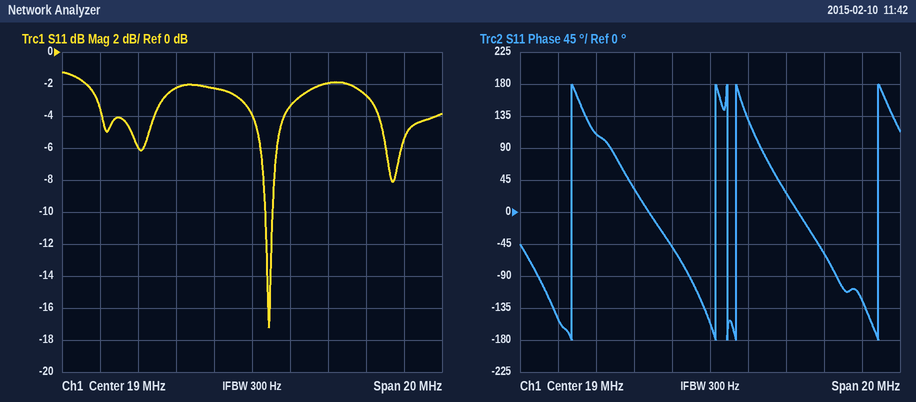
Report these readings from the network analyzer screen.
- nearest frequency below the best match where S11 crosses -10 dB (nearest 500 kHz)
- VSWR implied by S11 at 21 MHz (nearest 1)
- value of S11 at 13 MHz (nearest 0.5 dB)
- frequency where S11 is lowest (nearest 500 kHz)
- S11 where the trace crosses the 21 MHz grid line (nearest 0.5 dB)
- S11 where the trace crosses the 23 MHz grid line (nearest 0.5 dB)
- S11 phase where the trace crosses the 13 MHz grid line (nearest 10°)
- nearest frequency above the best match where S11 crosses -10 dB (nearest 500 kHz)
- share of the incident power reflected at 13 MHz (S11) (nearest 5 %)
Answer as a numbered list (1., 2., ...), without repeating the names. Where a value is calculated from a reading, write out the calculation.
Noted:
1. 19.5 MHz
2. |Γ| = 10^(-3.5/20) = 0.6683; VSWR = (1 + 0.6683)/(1 − 0.6683) ≈ 5
3. -6.0 dB
4. 20.0 MHz
5. -3.5 dB
6. -2.0 dB
7. 110°
8. 20.0 MHz
9. 10^(-6/10) ≈ 25 %
